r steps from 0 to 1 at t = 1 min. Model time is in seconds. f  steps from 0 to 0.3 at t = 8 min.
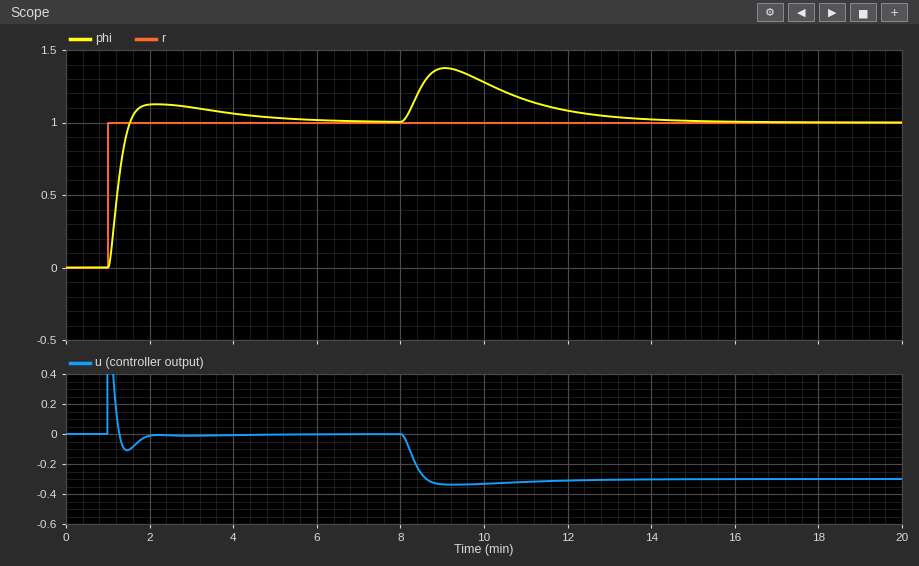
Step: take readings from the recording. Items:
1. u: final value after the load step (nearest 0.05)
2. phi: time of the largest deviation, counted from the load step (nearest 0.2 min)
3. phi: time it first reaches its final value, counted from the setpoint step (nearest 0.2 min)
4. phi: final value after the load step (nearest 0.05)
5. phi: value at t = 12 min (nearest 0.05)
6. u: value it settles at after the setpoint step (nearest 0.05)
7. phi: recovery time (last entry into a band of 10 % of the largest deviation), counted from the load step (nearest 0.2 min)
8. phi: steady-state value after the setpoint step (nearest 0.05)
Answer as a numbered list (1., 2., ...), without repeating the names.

1. -0.30
2. 1.0 min
3. 0.6 min
4. 1.00
5. 1.10
6. 0.00
7. 5.2 min
8. 1.00
